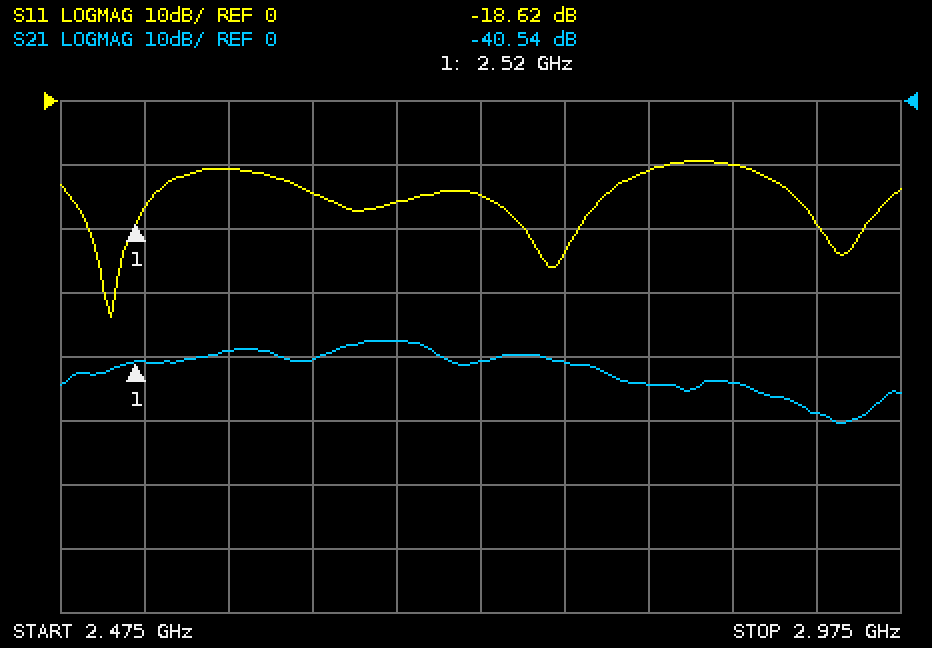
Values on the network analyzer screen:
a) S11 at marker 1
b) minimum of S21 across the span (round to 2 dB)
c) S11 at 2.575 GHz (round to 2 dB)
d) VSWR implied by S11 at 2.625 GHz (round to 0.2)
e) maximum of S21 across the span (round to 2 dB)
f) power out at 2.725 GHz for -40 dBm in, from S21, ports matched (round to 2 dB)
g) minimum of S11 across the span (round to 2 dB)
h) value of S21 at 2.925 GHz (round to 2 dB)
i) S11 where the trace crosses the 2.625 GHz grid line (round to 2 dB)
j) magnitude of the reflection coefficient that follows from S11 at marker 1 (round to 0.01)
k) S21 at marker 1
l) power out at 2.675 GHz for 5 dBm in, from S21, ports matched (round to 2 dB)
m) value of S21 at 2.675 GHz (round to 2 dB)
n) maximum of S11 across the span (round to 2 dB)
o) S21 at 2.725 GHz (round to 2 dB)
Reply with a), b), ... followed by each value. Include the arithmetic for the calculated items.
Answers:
a) -18.62 dB
b) -50 dB
c) -10 dB
d) |Γ| = 10^(-14/20) = 0.1995; VSWR = (1 + 0.1995)/(1 − 0.1995) ≈ 1.50, so 1.4 to the nearest 0.2
e) -38 dB
f) -40 dBm + (-40 dB) = -80 dBm
g) -34 dB
h) -48 dB
i) -14 dB
j) 10^(-18.62/20) ≈ 0.12
k) -40.54 dB
l) 5 dBm + (-38 dB) = -32 dBm
m) -38 dB
n) -10 dB
o) -40 dB
